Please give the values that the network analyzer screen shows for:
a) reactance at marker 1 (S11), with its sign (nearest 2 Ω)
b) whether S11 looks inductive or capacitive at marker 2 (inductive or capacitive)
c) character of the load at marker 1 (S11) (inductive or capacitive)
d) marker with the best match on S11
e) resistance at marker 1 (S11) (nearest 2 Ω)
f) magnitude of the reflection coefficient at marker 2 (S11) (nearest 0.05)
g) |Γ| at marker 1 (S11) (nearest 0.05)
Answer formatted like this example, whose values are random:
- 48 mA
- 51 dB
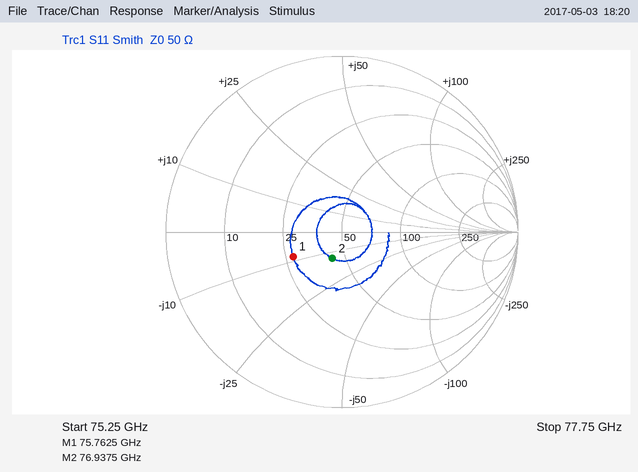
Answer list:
- -8 Ω
- capacitive
- capacitive
- marker 2
- 28 Ω
- 0.15
- 0.30
